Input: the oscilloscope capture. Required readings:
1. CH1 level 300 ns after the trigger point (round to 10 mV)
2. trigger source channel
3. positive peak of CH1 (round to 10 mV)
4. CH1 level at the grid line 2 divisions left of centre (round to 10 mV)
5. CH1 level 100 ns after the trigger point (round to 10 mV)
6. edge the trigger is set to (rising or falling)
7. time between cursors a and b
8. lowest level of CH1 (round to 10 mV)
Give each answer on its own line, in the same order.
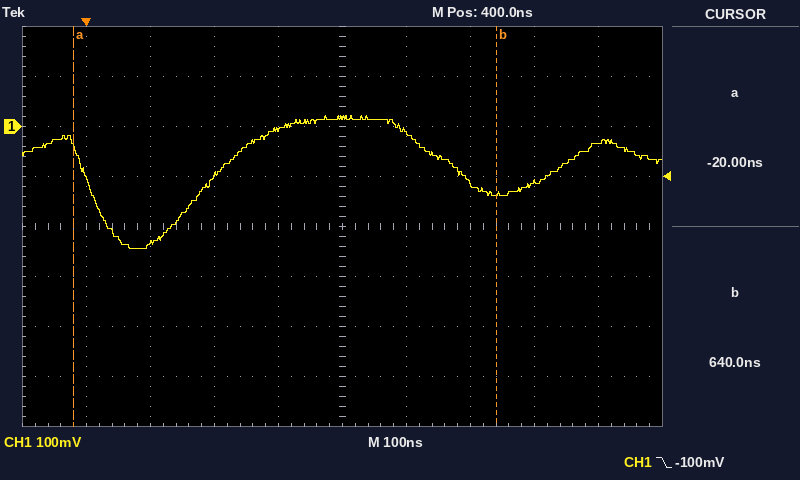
-10 mV
CH1
20 mV
-100 mV
-230 mV
falling
660 ns
-240 mV
